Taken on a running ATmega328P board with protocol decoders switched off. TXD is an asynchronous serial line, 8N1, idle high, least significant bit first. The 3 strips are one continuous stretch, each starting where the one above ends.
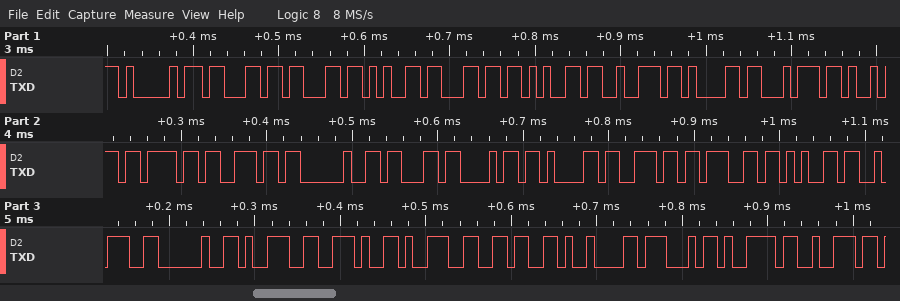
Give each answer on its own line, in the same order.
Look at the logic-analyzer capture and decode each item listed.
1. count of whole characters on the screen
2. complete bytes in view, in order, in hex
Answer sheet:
29
41 63 63 65 6C 65 72 61 74 69 6F 6E 20 63 68 61 6E 67 65 3A 20 39 2E 39 36 09 47 79 72
